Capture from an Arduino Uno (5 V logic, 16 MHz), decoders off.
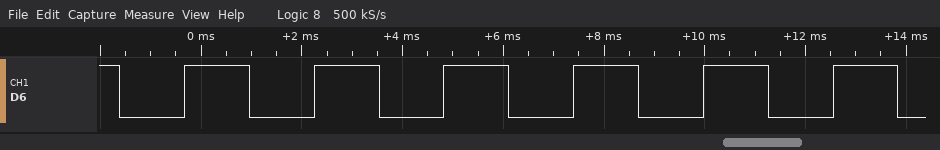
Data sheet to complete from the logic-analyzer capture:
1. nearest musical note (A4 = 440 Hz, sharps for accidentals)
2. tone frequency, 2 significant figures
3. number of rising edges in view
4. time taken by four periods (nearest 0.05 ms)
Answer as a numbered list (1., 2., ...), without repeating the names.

1. G4
2. 390 Hz
3. 6
4. 10.30 ms
